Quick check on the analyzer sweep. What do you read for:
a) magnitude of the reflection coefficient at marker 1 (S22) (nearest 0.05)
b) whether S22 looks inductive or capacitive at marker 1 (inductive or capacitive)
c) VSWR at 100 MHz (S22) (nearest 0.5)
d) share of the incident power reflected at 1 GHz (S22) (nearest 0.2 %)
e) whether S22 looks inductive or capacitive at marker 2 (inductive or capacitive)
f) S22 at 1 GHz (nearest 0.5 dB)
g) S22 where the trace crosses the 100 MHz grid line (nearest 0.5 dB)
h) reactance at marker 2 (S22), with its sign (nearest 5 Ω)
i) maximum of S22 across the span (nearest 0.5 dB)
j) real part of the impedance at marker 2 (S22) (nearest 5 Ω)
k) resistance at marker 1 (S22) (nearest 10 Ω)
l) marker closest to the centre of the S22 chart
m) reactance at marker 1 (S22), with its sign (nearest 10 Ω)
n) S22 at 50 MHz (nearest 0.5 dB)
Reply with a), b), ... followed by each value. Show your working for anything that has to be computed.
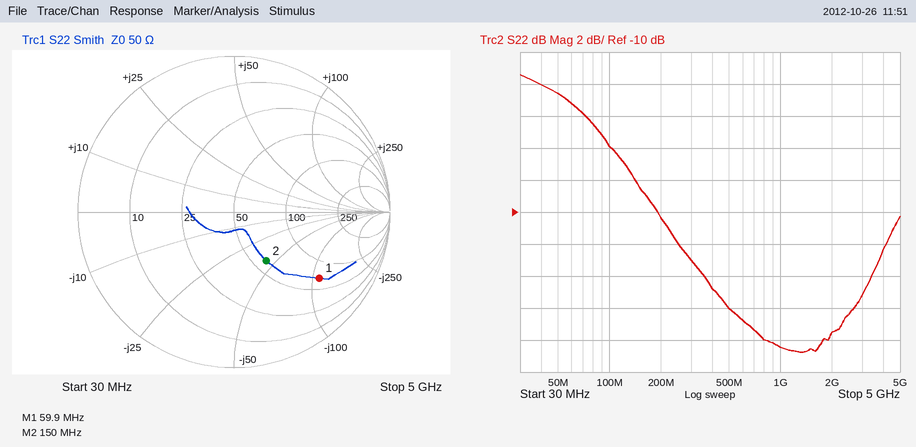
a) 0.70
b) capacitive
c) |Γ| = 10^(-6/20) = 0.5012; VSWR = (1 + 0.5012)/(1 − 0.5012) ≈ 3.0
d) 10^(-18.5/10) ≈ 1.4 %
e) capacitive
f) -18.5 dB
g) -6.0 dB
h) -45 Ω
i) -1.5 dB
j) 60 Ω
k) 70 Ω
l) marker 2
m) -110 Ω
n) -2.5 dB
